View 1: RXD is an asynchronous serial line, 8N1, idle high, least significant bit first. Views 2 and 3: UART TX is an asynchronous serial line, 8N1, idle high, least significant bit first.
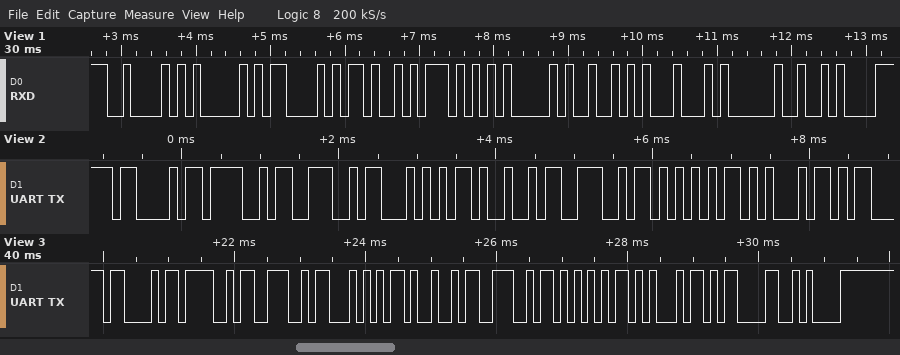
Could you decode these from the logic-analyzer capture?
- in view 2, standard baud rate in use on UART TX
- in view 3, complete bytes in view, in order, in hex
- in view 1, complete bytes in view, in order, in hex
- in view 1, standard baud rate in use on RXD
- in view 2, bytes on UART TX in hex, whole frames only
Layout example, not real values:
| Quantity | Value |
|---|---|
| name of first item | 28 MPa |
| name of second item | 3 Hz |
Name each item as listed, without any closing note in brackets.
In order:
| Quantity | Value |
|---|---|
| in view 2, standard baud rate in use on UART TX | 9600 baud |
| in view 3, complete bytes in view, in order, in hex | 43 4F 4E 54 49 4E 55 45 0D 0A |
| in view 1, complete bytes in view, in order, in hex | 0x42 0x41 0x43 0x4B 0x57 0x41 0x52 0x44 0x20 0x0A |
| in view 1, standard baud rate in use on RXD | 9600 baud |
| in view 2, bytes on UART TX in hex, whole frames only | 43 4F 4E 54 49 4E 55 45 |
